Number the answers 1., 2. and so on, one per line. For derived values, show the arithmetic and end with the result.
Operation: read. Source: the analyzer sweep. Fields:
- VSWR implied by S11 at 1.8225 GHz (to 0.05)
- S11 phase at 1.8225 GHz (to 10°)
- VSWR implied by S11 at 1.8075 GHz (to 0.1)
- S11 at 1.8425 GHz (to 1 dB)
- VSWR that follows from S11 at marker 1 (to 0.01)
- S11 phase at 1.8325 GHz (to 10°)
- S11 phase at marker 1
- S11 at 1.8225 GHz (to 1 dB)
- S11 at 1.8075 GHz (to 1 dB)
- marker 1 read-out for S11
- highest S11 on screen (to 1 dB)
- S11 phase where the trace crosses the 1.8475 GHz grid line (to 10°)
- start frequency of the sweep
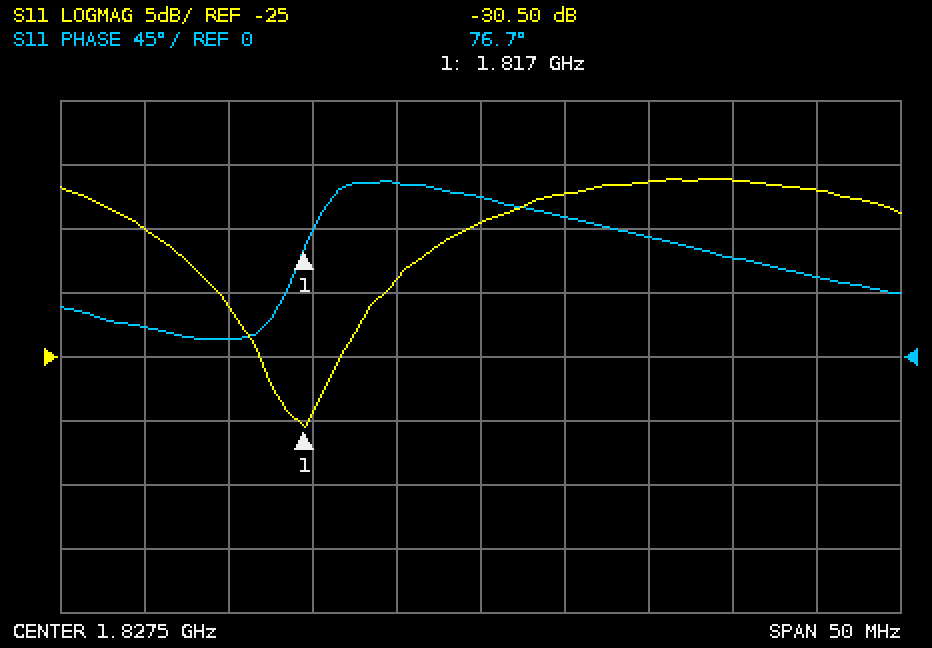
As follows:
1. |Γ| = 10^(-19/20) = 0.1122; VSWR = (1 + 0.1122)/(1 − 0.1122) ≈ 1.25
2. 120°
3. |Γ| = 10^(-15/20) = 0.1778; VSWR = (1 + 0.1778)/(1 − 0.1778) ≈ 1.4
4. -11 dB
5. (1 + 0.0299)/(1 − 0.0299) ≈ 1.06
6. 100°
7. 76.7°
8. -19 dB
9. -15 dB
10. -30.50 dB
11. -11 dB
12. 60°
13. 1.8025 GHz
